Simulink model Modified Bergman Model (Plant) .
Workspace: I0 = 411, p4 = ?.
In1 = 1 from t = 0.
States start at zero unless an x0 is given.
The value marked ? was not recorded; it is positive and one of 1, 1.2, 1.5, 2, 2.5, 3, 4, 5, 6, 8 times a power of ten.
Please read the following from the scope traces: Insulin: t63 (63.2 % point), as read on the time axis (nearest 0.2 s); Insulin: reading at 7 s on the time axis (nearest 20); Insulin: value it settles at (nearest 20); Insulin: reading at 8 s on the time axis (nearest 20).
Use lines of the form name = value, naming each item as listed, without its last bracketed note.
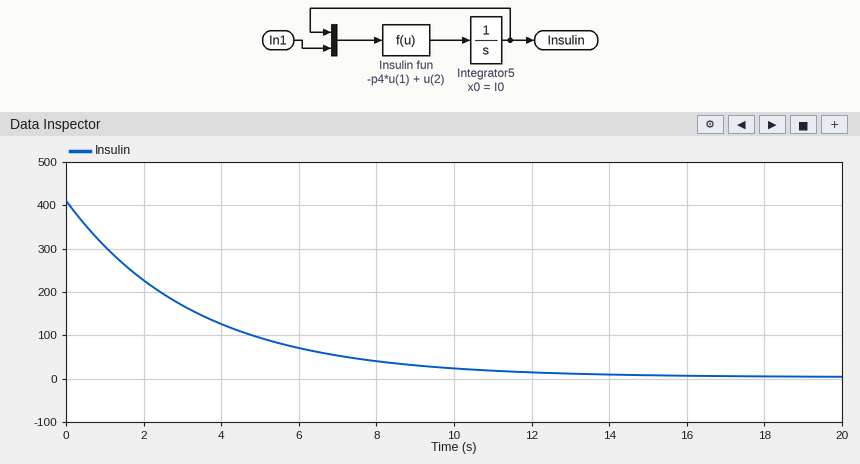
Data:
Insulin: t63 (63.2 % point), as read on the time axis = 3.4 s
Insulin: reading at 7 s on the time axis = 60
Insulin: value it settles at = 0
Insulin: reading at 8 s on the time axis = 40
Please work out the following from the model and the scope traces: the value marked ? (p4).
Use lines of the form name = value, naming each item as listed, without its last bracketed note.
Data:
the value marked ? = 0.3
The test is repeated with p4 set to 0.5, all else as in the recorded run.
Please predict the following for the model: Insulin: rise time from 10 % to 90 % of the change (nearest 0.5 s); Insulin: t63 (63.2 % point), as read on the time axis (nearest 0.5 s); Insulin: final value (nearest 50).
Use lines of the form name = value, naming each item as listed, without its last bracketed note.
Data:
Insulin: rise time from 10 % to 90 % of the change = 4.5 s
Insulin: t63 (63.2 % point), as read on the time axis = 2.0 s
Insulin: final value = 0
